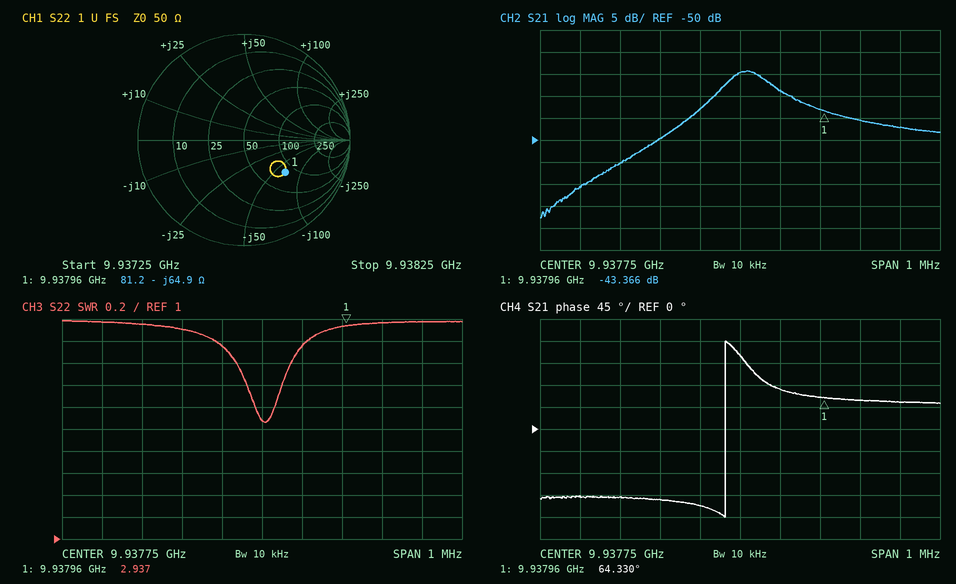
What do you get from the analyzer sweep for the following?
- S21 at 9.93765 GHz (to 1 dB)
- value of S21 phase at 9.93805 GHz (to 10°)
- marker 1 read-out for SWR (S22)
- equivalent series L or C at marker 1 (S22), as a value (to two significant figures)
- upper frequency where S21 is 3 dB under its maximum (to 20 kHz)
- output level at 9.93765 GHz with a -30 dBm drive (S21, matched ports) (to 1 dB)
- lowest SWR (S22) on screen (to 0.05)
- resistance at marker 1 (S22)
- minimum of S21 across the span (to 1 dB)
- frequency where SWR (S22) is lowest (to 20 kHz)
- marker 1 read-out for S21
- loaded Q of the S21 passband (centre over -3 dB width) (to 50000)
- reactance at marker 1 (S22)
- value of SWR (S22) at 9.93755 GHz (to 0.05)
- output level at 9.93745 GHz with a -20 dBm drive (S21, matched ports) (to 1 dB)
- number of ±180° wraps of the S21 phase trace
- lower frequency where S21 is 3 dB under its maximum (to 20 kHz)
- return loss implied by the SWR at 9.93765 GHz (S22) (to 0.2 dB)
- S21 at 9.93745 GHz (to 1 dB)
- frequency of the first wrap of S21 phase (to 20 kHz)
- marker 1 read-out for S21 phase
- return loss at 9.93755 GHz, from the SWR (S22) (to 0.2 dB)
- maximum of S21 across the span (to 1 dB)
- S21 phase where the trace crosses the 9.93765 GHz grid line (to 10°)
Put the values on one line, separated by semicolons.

-43 dB; 60°; 2.937; 250 fF; 9.93782 GHz; -73 dBm; 2.05; 81.2 Ω; -68 dB; 9.93776 GHz; -43.366 dB; 100000; -64.9 Ω; 2.90; -75 dBm; 1; 9.93772 GHz; 6.6 dB; -55 dB; 9.93772 GHz; 64.330°; 6.2 dB; -34 dB; -160°
